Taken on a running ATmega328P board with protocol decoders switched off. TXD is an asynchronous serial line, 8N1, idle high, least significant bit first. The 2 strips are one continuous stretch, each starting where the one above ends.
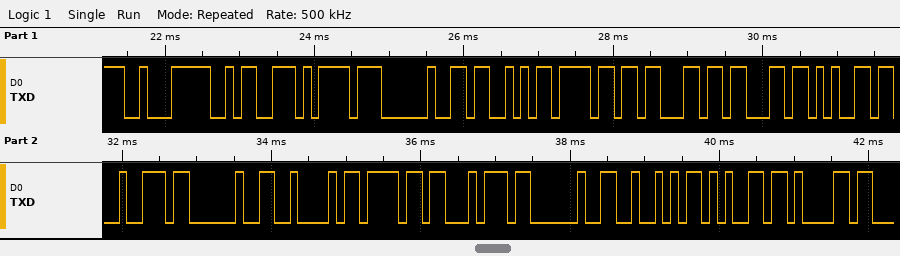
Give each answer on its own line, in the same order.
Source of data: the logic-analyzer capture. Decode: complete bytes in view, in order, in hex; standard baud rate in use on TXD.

0xE2 0x9A 0xBD 0x20 0x53 0x6F 0x63 0x63 0x65 0x72 0x20 0x42 0x6F 0x74 0x20 0x52 0x65 0x61
9600 baud
